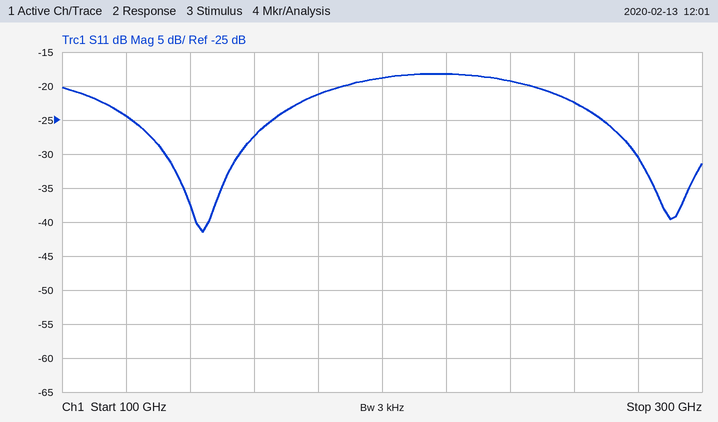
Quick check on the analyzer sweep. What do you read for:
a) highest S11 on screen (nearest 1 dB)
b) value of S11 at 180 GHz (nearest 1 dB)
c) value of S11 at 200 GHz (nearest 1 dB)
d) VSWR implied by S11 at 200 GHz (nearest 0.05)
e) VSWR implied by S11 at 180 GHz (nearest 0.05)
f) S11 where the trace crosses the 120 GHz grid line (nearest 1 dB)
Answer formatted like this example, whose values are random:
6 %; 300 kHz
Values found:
-18 dB; -21 dB; -19 dB; 1.25; 1.20; -24 dB
